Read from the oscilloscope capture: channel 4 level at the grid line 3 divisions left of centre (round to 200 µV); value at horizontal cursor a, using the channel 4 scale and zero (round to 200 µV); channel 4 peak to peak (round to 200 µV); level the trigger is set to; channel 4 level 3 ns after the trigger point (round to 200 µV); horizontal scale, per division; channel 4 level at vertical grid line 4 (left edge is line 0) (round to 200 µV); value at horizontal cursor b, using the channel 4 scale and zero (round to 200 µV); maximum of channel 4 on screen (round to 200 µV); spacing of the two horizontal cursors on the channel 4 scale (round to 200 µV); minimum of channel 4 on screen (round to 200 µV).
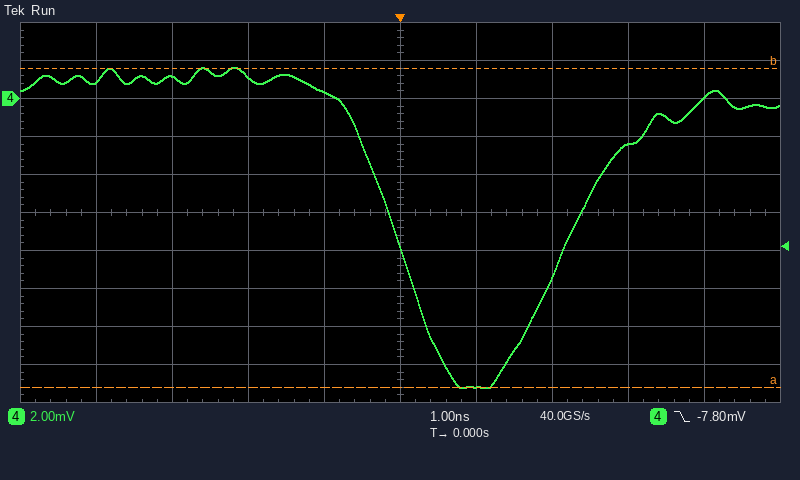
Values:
1.2 mV
-15.2 mV
16.8 mV
-7.80 mV
-2.4 mV
1 ns
400 µV
1.6 mV
1.6 mV
16.8 mV
-15.2 mV
